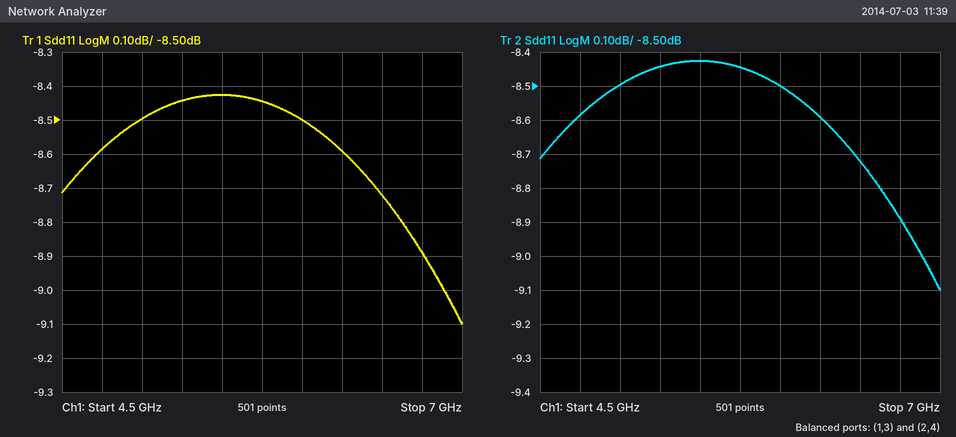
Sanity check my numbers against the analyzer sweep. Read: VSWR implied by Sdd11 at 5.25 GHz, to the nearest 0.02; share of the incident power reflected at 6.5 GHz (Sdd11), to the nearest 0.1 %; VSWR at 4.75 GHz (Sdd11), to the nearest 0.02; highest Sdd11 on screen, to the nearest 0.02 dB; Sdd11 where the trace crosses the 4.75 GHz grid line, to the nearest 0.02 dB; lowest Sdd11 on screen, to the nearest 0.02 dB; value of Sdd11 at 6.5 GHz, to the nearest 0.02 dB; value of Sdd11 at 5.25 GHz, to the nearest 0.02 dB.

2.22
13.4 %
2.18
-8.42 dB
-8.58 dB
-9.10 dB
-8.72 dB
-8.44 dB
